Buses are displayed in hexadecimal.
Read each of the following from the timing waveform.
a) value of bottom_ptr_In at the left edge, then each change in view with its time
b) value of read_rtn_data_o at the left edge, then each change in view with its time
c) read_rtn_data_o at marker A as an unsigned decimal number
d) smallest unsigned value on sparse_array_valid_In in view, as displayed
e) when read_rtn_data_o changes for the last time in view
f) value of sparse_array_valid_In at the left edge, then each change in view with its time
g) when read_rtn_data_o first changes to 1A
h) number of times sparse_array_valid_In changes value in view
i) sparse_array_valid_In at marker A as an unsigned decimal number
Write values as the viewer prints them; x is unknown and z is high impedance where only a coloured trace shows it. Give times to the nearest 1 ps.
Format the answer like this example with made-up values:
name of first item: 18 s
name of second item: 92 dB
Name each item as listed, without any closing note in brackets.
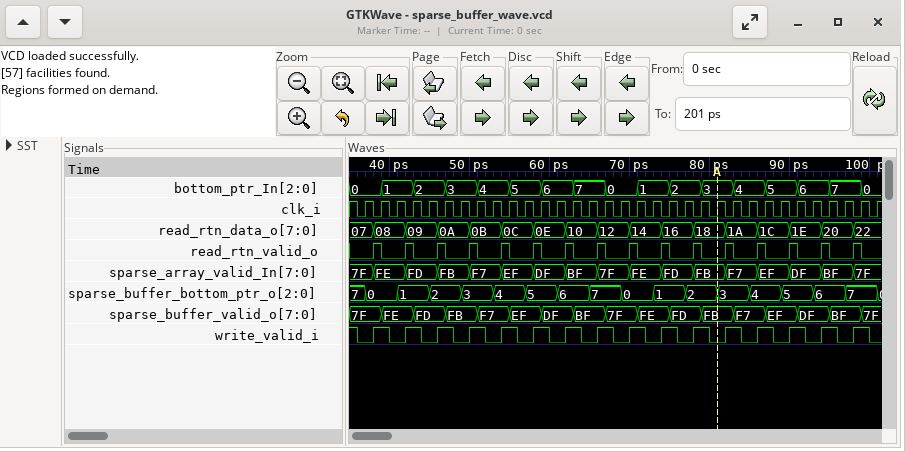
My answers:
value of bottom_ptr_In at the left edge, then each change in view with its time: 0, 1 at 39 ps, 2 at 43 ps, 3 at 47 ps, 4 at 51 ps, 5 at 55 ps, 6 at 59 ps, 7 at 63 ps, 0 at 67 ps, 1 at 71 ps, 2 at 75 ps, 3 at 79 ps, 4 at 83 ps, 5 at 87 ps, 6 at 91 ps, 7 at 95 ps, 0 at 99 ps
value of read_rtn_data_o at the left edge, then each change in view with its time: 07, 08 at 38 ps, 09 at 42 ps, 0A at 46 ps, 0B at 50 ps, 0C at 54 ps, 0E at 58 ps, 10 at 62 ps, 12 at 66 ps, 14 at 70 ps, 16 at 74 ps, 18 at 78 ps, 1A at 82 ps, 1C at 86 ps, 1E at 90 ps, 20 at 94 ps, 22 at 98 ps
read_rtn_data_o at marker A as an unsigned decimal number: 24
smallest unsigned value on sparse_array_valid_In in view, as displayed: 7F
when read_rtn_data_o changes for the last time in view: 98 ps
value of sparse_array_valid_In at the left edge, then each change in view with its time: 7F, FE at 38 ps, FD at 42 ps, FB at 46 ps, F7 at 50 ps, EF at 54 ps, DF at 58 ps, BF at 62 ps, 7F at 66 ps, FE at 70 ps, FD at 74 ps, FB at 78 ps, F7 at 82 ps, EF at 86 ps, DF at 90 ps, BF at 94 ps, 7F at 98 ps
when read_rtn_data_o first changes to 1A: 82 ps
number of times sparse_array_valid_In changes value in view: 16
sparse_array_valid_In at marker A as an unsigned decimal number: 251
